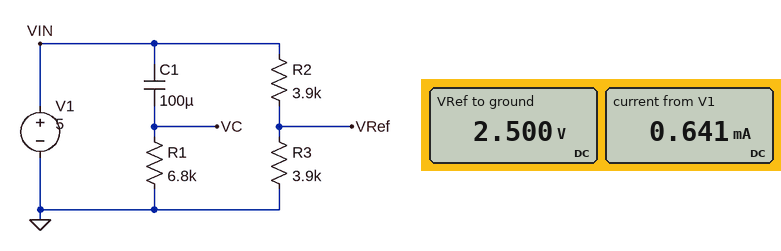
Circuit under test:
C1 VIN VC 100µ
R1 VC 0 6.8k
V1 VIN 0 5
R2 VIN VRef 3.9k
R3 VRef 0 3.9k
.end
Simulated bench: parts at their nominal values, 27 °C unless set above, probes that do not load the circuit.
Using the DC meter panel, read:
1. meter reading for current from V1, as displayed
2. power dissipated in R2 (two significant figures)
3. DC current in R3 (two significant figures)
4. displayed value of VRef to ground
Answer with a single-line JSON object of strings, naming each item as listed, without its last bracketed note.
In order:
{"meter reading for current from V1, as displayed": "0.641 mA", "power dissipated in R2": "1.6 mW", "DC current in R3": "640 µA", "displayed value of VRef to ground": "2.500 V"}
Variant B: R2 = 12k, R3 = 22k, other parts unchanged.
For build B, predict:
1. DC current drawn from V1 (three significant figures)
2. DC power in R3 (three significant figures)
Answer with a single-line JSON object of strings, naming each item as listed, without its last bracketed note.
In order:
{"DC current drawn from V1": "147 µA", "DC power in R3": "476 µW"}
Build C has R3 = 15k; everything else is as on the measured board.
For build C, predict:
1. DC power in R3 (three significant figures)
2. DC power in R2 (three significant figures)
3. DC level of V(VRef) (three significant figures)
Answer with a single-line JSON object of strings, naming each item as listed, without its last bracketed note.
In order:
{"DC power in R3": "1.05 mW", "DC power in R2": "273 µW", "DC level of V(VRef)": "3.97 V"}
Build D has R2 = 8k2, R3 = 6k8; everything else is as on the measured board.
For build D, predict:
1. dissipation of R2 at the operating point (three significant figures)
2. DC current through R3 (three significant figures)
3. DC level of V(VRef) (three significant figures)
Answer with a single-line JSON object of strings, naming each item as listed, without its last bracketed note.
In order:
{"dissipation of R2 at the operating point": "911 µW", "DC current through R3": "333 µA", "DC level of V(VRef)": "2.27 V"}
